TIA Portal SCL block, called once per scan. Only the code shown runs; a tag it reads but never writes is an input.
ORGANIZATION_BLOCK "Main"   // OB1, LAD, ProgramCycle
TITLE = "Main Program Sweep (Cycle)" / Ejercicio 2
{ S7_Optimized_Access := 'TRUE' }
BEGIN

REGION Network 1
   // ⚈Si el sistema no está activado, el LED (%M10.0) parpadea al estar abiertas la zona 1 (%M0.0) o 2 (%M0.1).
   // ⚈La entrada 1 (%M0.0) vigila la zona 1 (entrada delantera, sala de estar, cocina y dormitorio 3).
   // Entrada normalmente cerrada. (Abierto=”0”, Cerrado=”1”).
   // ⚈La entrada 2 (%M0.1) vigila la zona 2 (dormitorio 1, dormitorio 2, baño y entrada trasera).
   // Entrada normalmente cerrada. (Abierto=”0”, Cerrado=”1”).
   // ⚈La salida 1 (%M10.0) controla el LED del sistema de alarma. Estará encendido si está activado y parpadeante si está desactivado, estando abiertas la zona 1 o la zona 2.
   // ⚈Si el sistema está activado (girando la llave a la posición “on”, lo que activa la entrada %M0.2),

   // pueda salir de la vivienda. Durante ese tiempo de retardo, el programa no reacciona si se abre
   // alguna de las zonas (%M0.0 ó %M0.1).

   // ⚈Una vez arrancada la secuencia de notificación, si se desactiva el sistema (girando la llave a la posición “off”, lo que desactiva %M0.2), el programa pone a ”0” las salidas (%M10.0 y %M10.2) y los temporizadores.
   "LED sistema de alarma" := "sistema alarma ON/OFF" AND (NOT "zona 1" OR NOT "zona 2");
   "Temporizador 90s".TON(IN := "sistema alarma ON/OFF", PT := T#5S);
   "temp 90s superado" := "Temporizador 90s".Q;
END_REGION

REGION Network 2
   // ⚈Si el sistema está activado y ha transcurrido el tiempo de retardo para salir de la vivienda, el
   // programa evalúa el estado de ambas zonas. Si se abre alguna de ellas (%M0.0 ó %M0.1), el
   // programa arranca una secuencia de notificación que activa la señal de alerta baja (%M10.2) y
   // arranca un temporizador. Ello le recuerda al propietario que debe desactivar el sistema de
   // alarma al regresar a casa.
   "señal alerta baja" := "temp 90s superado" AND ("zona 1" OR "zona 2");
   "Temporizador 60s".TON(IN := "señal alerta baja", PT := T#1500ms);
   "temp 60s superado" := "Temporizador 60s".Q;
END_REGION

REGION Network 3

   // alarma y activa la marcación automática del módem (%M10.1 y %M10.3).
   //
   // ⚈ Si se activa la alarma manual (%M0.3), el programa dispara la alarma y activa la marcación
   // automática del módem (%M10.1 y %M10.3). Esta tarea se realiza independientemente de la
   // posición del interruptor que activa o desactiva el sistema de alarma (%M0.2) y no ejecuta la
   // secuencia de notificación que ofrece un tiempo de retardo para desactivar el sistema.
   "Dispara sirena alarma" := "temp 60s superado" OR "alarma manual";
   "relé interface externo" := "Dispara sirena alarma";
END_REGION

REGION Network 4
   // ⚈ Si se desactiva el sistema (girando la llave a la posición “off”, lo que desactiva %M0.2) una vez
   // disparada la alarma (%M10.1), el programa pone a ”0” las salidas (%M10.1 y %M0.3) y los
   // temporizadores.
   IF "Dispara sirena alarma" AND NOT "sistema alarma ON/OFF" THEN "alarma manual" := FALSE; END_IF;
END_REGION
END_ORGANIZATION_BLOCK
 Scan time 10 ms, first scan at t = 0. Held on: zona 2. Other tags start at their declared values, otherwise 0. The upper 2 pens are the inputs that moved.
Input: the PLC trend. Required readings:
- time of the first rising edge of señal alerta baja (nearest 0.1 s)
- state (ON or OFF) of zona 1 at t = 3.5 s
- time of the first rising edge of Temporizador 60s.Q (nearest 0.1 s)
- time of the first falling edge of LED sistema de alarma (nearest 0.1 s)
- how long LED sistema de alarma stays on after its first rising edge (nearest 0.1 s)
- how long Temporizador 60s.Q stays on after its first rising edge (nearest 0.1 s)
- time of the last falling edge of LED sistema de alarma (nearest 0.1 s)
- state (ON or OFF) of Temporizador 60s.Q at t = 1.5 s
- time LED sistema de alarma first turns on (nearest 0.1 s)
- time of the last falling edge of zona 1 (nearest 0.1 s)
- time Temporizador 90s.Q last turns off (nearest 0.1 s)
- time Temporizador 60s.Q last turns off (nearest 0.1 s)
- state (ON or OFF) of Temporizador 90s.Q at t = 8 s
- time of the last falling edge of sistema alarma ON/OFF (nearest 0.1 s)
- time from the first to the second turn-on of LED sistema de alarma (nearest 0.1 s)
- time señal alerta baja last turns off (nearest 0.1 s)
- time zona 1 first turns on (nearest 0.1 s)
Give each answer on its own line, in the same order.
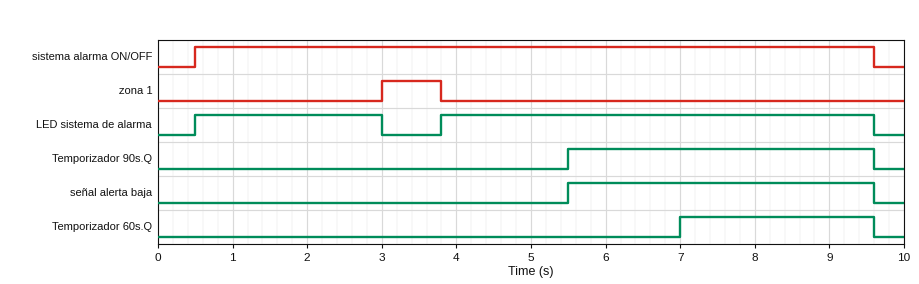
5.5 s
ON
7.0 s
3.0 s
2.5 s
2.6 s
9.6 s
OFF
0.5 s
3.8 s
9.6 s
9.6 s
ON
9.6 s
3.3 s
9.6 s
3.0 s
